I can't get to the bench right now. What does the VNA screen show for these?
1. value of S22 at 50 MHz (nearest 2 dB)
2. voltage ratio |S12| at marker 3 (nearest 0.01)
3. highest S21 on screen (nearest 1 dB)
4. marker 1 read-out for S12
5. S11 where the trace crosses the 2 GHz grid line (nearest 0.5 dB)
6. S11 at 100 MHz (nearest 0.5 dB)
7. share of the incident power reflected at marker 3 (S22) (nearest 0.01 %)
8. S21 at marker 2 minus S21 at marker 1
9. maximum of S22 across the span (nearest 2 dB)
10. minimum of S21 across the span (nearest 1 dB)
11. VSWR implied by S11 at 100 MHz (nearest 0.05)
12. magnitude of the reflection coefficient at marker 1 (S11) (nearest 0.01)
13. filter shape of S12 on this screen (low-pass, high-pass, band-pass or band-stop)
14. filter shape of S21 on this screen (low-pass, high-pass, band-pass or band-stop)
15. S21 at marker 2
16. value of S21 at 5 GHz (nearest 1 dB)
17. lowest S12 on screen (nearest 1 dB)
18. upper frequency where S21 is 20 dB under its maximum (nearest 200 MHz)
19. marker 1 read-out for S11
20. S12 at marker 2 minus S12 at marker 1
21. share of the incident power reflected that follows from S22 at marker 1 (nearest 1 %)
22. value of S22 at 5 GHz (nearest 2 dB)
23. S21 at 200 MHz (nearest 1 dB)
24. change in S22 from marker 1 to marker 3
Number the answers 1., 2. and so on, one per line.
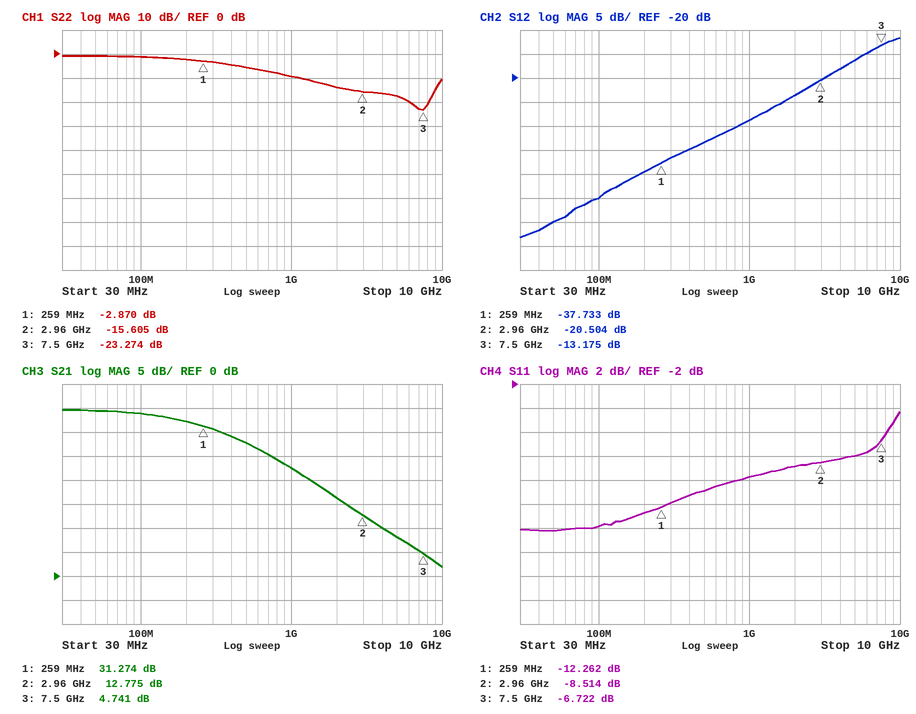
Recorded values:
1. 0 dB
2. 0.22
3. 35 dB
4. -37.733 dB
5. -9.0 dB
6. -14.0 dB
7. 0.47 %
8. -18.499 dB
9. 0 dB
10. 2 dB
11. 1.50
12. 0.24
13. high-pass
14. low-pass
15. 12.775 dB
16. 8 dB
17. -53 dB
18. 2.4 GHz
19. -12.262 dB
20. 17.229 dB
21. 52 %
22. -18 dB
23. 32 dB
24. -20.404 dB
